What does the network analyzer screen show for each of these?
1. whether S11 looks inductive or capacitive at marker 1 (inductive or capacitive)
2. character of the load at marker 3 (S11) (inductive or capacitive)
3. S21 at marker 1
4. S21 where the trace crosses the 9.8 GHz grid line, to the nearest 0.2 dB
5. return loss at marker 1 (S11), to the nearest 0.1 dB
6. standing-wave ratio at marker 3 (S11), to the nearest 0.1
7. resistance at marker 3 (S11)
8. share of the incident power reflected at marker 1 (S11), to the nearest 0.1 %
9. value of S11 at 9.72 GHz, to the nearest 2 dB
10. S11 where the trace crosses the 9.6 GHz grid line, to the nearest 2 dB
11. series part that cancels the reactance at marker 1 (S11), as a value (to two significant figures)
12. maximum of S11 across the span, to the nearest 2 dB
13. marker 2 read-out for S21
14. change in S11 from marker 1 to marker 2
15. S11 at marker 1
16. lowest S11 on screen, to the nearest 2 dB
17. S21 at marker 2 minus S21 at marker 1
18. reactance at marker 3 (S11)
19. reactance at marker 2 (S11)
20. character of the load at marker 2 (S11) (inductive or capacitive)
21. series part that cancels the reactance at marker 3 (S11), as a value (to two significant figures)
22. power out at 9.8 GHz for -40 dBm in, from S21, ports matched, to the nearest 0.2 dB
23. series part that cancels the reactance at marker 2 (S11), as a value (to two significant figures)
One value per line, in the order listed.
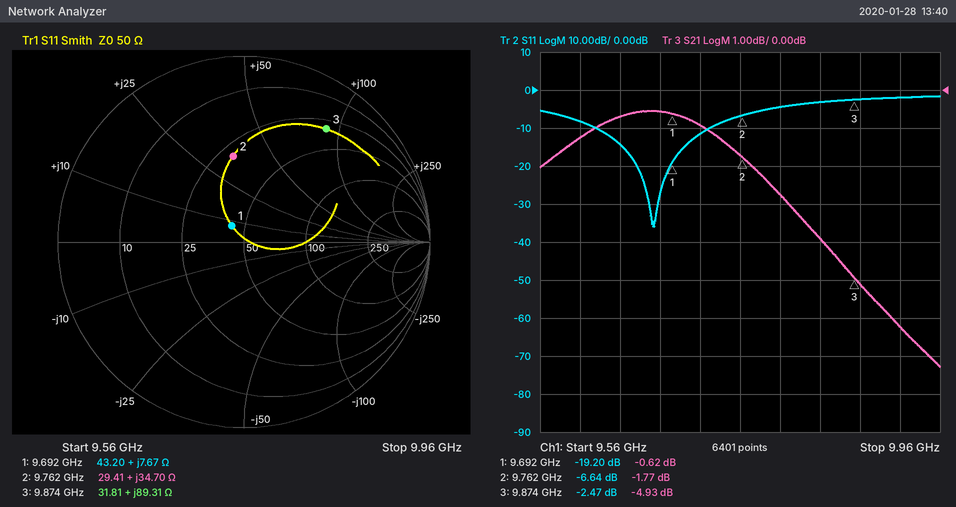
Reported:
inductive
inductive
-0.62 dB
-2.8 dB
19.2 dB
7.1
31.81 Ω
1.2 %
-12 dB
-8 dB
2.1 pF
-2 dB
-1.77 dB
12.56 dB
-19.20 dB
-36 dB
-1.15 dB
+89.31 Ω
+34.70 Ω
inductive
180 fF
-42.8 dBm
470 fF
